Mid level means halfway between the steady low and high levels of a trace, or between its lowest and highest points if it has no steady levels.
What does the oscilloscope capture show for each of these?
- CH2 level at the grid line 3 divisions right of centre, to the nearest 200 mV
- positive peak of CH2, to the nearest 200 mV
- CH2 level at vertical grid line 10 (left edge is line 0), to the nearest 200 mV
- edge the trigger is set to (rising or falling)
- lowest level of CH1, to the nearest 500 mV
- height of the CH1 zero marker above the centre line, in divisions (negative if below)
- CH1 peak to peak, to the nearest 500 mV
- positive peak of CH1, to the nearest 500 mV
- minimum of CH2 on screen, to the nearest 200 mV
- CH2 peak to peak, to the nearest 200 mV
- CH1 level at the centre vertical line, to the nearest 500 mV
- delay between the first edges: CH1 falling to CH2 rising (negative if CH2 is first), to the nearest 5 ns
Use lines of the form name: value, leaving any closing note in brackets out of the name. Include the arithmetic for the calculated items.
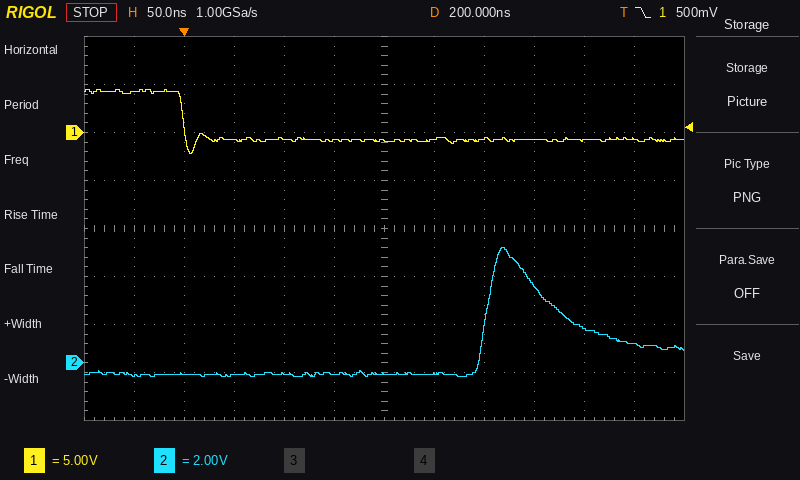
CH2 level at the grid line 3 divisions right of centre, to the nearest 200 mV: 3.2 V
positive peak of CH2, to the nearest 200 mV: 4.8 V
CH2 level at vertical grid line 10 (left edge is line 0), to the nearest 200 mV: 1.4 V
edge the trigger is set to: falling
lowest level of CH1, to the nearest 500 mV: -2.0 V
height of the CH1 zero marker above the centre line, in divisions: +2.0 div
CH1 peak to peak, to the nearest 500 mV: 4.5 V − (-2.0 V) = 6.5 V
positive peak of CH1, to the nearest 500 mV: 4.5 V
minimum of CH2 on screen, to the nearest 200 mV: -600 mV
CH2 peak to peak, to the nearest 200 mV: 4.8 V − (-600 mV) = 5.4 V
CH1 level at the centre vertical line, to the nearest 500 mV: -1.0 V
delay between the first edges: CH1 falling to CH2 rising (negative if CH2 is first), to the nearest 5 ns: +305 ns
